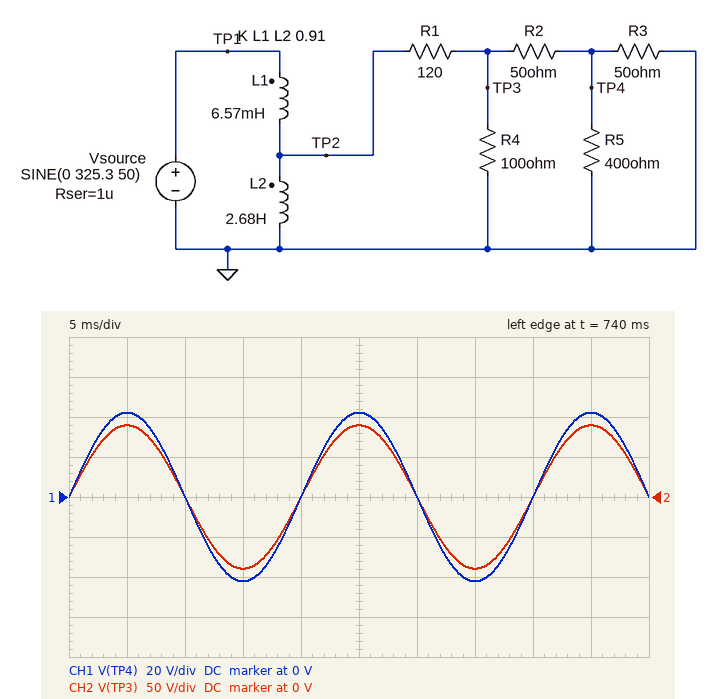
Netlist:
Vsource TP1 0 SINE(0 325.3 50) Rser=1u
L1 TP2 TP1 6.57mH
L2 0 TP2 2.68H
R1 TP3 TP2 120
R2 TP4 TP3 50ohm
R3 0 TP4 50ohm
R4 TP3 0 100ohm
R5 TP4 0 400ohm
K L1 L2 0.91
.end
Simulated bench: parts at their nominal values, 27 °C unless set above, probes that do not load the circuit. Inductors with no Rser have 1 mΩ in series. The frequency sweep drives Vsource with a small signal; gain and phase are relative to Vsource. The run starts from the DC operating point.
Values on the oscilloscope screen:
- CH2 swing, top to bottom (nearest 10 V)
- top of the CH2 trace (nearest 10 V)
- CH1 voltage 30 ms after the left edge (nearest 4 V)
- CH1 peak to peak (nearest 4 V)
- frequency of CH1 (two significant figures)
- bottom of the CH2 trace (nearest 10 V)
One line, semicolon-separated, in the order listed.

180 V; 90 V; 0 V; 84 V; 50 Hz; -90 V
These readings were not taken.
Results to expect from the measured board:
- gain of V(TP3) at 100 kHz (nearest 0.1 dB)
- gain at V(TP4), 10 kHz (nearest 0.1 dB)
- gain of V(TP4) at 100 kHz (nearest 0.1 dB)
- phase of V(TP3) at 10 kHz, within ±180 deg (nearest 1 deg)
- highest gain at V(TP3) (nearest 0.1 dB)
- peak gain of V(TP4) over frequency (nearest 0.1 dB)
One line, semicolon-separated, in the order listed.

-23.2 dB; -18.3 dB; -29.7 dB; -21 deg; -11.2 dB; -17.7 dB
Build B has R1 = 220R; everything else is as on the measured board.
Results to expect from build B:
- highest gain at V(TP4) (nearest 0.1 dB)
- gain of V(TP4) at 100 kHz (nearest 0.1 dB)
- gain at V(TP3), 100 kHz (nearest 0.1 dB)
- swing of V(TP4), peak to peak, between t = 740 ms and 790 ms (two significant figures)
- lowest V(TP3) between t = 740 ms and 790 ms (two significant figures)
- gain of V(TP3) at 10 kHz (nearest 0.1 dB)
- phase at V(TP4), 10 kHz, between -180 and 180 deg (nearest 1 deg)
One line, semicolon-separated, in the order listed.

-21.8 dB; -30.1 dB; -23.6 dB; 53 V; -56 V; -15.5 dB; -14 deg
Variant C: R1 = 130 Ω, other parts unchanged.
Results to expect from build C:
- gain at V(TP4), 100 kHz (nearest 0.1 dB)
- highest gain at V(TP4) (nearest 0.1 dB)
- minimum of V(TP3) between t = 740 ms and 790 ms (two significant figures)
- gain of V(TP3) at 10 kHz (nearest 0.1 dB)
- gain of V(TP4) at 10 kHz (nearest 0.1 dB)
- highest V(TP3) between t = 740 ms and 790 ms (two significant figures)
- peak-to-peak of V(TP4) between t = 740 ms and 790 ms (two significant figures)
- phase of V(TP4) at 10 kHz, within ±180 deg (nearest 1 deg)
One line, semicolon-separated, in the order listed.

-29.8 dB; -18.2 dB; -85 V; -12.2 dB; -18.8 dB; 85 V; 80 V; -20 deg
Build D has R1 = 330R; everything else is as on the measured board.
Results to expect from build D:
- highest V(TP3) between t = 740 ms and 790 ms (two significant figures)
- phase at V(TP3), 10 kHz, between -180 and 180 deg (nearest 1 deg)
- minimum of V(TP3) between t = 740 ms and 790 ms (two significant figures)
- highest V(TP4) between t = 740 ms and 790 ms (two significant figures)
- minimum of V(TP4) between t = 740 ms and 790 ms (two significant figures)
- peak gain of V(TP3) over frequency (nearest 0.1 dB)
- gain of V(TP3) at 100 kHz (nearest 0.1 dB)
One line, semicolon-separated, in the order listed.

40 V; -10 deg; -40 V; 19 V; -19 V; -18.2 dB; -24.2 dB
